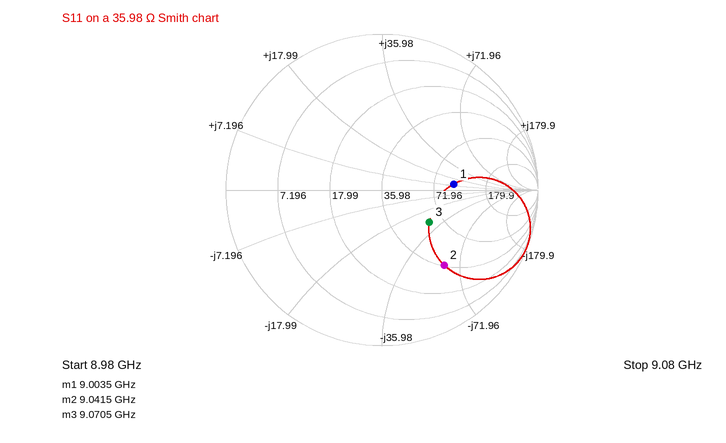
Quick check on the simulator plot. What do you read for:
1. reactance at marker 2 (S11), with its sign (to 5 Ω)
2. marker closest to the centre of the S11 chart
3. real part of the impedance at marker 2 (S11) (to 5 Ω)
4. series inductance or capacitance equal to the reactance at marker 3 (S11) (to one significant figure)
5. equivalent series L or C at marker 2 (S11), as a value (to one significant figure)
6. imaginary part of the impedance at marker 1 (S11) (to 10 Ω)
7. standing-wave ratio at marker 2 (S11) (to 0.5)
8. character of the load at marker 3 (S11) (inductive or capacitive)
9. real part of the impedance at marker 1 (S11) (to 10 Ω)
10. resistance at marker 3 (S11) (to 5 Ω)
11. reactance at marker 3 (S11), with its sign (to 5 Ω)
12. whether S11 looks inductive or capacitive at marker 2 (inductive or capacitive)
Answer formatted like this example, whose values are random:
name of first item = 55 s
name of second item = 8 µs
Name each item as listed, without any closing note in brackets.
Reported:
reactance at marker 2 (S11), with its sign = -60 Ω
marker closest to the centre of the S11 chart = marker 3
real part of the impedance at marker 2 (S11) = 35 Ω
series inductance or capacitance equal to the reactance at marker 3 (S11) = 600 fF
equivalent series L or C at marker 2 (S11), as a value = 300 fF
imaginary part of the impedance at marker 1 (S11) = +10 Ω
standing-wave ratio at marker 2 (S11) = 4.5
character of the load at marker 3 (S11) = capacitive
real part of the impedance at marker 1 (S11) = 100 Ω
resistance at marker 3 (S11) = 60 Ω
reactance at marker 3 (S11), with its sign = -30 Ω
whether S11 looks inductive or capacitive at marker 2 = capacitive
